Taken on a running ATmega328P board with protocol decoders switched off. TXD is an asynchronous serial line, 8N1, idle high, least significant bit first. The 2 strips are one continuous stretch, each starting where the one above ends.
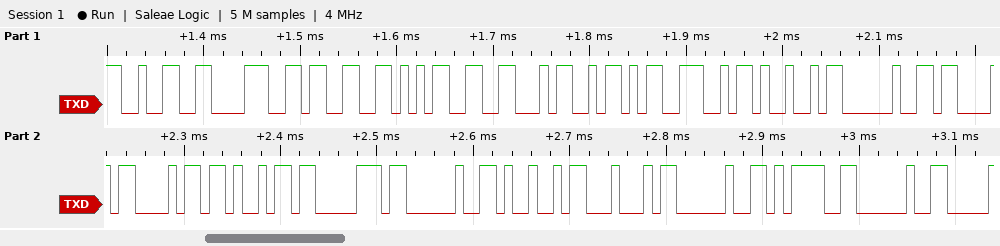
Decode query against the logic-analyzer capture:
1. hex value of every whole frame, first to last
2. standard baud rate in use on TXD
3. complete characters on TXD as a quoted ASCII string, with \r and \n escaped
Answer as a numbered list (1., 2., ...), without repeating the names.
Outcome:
1. 0x32 0x38 0x33 0x35 0x46 0x5A 0x4E 0x49 0x20 0x43 0x68 0x69 0x70 0x20 0x49 0x44 0x20 0x3D 0x20
2. 115200 baud
3. "2835FZNI Chip ID = "
